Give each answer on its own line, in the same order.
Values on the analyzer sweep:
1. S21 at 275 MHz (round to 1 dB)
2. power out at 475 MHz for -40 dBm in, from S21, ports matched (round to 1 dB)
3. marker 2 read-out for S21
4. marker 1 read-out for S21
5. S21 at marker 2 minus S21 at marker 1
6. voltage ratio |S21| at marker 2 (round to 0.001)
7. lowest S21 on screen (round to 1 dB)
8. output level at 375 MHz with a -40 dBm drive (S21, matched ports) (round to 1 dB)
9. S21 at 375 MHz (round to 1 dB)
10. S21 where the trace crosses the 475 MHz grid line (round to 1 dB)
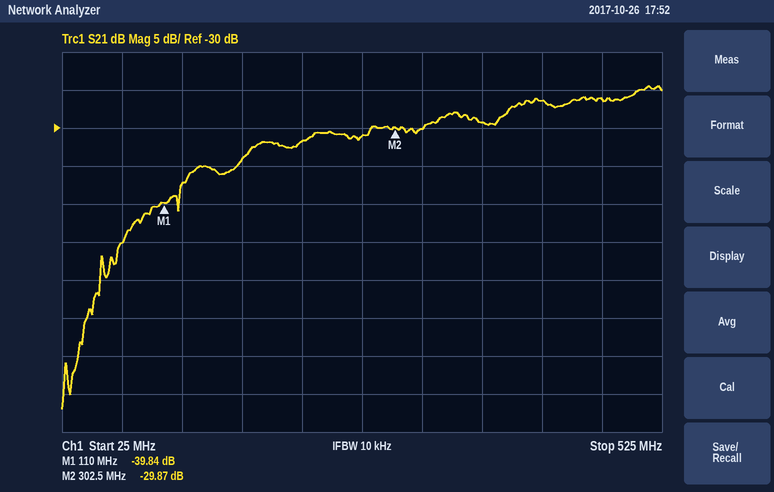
-31 dB
-66 dBm
-29.87 dB
-39.84 dB
9.97 dB
0.032
-67 dB
-69 dBm
-29 dB
-26 dB
